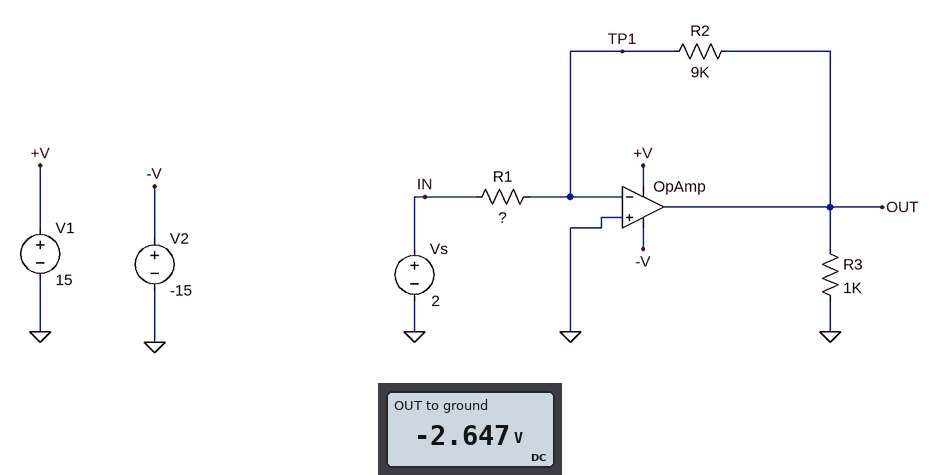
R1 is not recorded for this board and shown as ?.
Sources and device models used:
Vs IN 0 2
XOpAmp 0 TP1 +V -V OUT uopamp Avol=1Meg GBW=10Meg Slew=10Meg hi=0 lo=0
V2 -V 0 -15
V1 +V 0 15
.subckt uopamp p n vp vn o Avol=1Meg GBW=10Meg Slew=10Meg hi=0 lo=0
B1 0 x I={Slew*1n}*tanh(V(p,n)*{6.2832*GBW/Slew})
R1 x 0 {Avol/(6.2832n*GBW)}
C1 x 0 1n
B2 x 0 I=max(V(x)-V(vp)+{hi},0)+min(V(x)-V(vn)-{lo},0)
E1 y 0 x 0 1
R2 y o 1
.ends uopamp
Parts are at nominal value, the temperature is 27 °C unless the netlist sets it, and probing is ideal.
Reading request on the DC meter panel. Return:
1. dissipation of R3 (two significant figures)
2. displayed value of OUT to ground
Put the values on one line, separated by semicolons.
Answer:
7.0 mW; -2.647 V
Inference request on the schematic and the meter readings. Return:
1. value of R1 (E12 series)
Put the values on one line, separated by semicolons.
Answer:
6.8 kΩ
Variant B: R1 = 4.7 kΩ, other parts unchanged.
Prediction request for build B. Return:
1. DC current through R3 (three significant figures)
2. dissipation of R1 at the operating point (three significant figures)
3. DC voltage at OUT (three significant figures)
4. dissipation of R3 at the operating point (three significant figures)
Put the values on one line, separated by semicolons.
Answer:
3.83 mA; 851 µW; -3.83 V; 14.7 mW
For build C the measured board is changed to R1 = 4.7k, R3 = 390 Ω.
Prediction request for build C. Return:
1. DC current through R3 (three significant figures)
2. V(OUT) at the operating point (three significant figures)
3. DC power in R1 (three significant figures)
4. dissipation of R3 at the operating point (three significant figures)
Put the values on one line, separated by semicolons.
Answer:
9.82 mA; -3.83 V; 851 µW; 37.6 mW
